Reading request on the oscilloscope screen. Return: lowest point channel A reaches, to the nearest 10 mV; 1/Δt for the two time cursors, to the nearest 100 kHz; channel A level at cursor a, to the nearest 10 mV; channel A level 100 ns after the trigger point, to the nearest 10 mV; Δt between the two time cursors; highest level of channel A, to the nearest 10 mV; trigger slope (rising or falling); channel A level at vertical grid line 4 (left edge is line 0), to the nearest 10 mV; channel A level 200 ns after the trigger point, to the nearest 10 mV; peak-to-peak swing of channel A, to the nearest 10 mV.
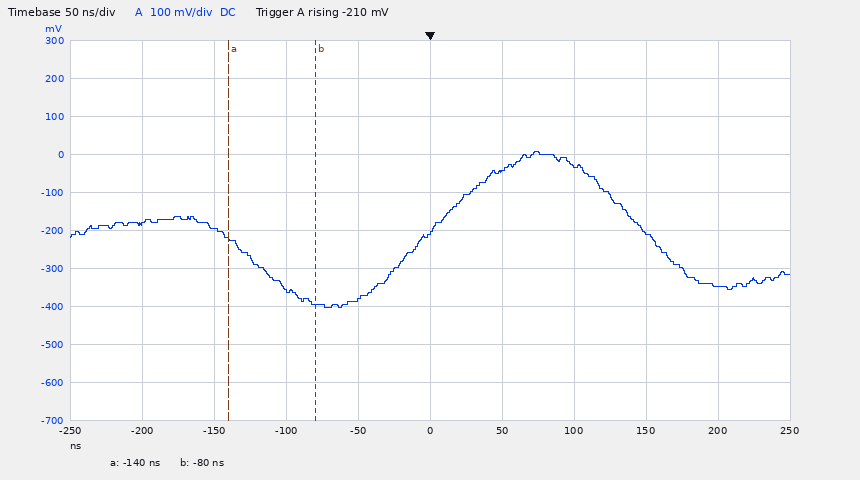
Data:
-400 mV
16.7 MHz
-220 mV
-30 mV
60 ns
10 mV
rising
-380 mV
-350 mV
410 mV
